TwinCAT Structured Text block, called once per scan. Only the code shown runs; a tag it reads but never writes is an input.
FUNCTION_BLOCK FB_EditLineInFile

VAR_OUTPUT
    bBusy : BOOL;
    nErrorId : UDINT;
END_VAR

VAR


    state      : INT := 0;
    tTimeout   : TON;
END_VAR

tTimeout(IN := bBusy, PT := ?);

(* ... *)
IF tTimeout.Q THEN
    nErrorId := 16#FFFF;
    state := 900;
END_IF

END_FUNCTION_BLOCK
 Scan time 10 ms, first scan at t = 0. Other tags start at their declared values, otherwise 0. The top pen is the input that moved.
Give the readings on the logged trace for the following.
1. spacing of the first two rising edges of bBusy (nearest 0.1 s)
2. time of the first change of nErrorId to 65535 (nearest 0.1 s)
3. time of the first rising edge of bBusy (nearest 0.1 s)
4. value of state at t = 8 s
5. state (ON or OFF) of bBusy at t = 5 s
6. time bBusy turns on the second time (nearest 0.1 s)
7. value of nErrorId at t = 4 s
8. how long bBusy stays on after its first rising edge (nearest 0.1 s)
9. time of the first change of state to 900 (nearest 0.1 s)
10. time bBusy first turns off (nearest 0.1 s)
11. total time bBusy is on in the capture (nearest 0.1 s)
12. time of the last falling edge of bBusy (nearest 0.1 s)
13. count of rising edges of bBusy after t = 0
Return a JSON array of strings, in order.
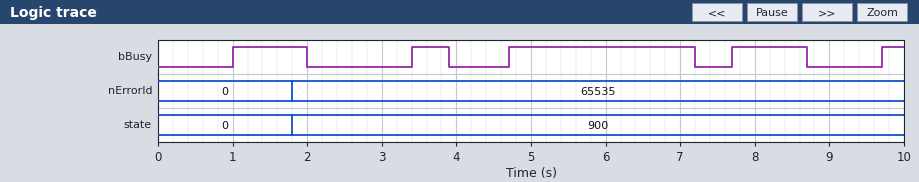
["2.4 s", "1.8 s", "1.0 s", "900", "ON", "3.4 s", "65535", "1.0 s", "1.8 s", "2.0 s", "5.3 s", "8.7 s", "5"]
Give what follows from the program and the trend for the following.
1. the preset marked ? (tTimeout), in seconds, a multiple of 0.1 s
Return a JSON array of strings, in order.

["0.8 s"]
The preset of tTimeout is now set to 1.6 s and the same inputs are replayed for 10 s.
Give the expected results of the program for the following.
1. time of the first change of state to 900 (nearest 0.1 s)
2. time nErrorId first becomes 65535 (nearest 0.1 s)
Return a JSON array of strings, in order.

["6.3 s", "6.3 s"]
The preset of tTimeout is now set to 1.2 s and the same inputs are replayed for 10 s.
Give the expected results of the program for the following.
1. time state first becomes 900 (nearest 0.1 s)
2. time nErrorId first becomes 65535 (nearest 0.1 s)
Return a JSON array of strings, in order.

["5.9 s", "5.9 s"]
